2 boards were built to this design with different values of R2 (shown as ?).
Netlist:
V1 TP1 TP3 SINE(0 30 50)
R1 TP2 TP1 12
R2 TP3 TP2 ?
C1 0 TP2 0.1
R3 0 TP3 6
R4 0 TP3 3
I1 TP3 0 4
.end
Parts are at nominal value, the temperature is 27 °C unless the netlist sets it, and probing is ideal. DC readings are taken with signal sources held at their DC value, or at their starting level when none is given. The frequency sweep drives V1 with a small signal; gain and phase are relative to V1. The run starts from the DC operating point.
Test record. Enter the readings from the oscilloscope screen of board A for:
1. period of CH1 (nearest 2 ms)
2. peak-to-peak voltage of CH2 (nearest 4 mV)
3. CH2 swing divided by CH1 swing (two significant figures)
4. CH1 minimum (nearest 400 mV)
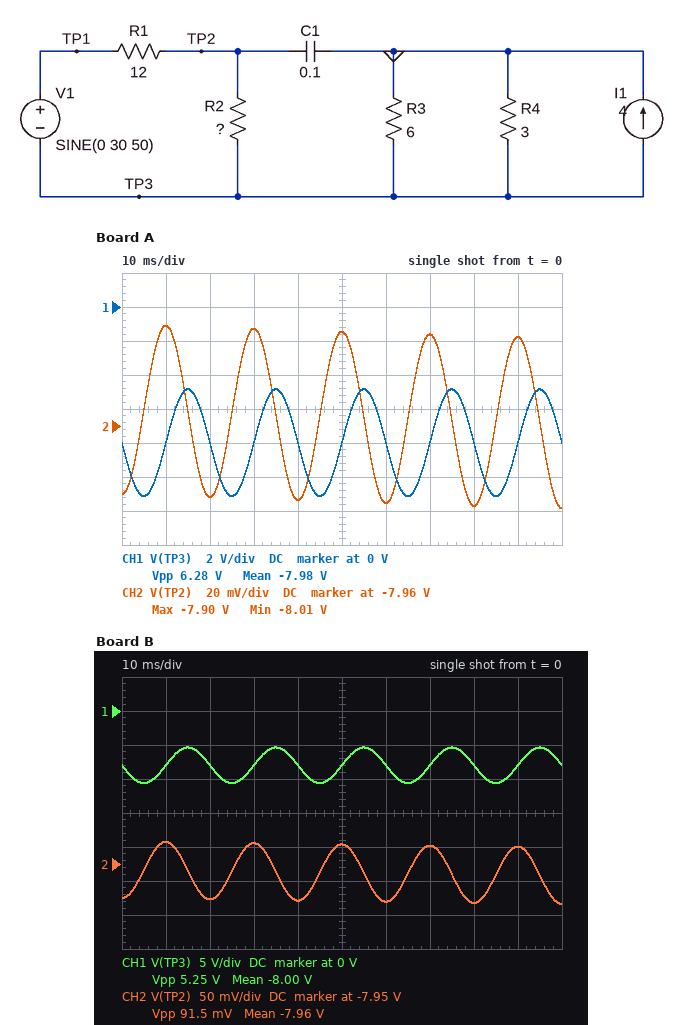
20 ms
108 mV
0.017
-11.2 V
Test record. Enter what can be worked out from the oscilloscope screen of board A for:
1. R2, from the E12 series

4.7 Ω
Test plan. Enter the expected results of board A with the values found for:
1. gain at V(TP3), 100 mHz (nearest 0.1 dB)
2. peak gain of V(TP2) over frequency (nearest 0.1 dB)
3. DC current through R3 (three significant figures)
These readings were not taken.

-29.5 dB
-11.0 dB
1.33 A
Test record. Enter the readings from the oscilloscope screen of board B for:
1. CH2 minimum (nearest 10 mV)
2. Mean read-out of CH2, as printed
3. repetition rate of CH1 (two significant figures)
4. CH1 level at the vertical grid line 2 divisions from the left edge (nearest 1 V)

-8.01 V
-7.96 V
50 Hz
-8 V
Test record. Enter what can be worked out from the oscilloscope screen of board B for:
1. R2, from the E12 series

2.7 Ω
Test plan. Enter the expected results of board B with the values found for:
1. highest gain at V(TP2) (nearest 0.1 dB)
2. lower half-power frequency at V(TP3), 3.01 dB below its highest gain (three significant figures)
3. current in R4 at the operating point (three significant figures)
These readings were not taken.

-14.7 dB
379 mHz
2.67 A
